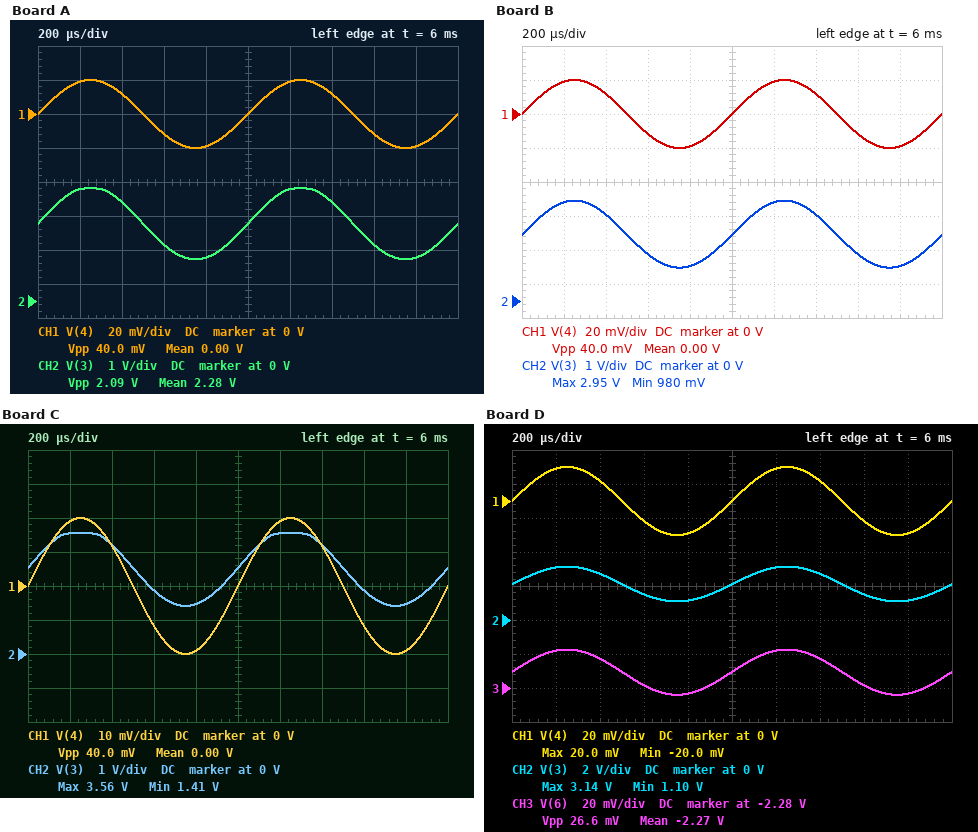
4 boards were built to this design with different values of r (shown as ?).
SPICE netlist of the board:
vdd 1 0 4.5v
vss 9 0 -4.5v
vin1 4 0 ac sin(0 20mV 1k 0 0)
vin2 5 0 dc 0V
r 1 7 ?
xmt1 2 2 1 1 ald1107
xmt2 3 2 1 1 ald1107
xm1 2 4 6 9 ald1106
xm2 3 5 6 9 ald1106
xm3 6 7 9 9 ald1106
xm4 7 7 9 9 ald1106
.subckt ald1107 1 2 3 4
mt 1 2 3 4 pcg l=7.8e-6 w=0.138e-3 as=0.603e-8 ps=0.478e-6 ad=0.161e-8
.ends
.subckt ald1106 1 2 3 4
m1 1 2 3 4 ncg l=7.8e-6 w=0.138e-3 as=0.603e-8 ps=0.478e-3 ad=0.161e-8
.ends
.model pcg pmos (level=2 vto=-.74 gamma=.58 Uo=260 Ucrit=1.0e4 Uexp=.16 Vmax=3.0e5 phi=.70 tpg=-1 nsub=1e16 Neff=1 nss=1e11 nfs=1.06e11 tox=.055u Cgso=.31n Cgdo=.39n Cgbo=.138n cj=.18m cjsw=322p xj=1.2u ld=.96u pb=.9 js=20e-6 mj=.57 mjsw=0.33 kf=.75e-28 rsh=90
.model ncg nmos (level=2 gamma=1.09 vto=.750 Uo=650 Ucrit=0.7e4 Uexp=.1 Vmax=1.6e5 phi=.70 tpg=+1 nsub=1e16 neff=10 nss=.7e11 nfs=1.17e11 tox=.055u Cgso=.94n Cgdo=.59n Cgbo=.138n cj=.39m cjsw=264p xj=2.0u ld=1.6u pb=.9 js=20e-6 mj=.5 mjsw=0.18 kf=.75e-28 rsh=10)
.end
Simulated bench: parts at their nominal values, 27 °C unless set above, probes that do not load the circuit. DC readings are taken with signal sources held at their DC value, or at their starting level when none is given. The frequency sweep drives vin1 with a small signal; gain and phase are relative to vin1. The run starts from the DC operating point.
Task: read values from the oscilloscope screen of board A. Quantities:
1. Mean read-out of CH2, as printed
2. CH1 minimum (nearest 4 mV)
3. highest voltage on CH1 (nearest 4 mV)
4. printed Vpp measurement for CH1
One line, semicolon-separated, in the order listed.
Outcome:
2.28 V; -20 mV; 20 mV; 40.0 mV
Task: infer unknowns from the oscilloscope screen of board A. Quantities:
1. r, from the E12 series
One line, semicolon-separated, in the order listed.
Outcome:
15 kΩ
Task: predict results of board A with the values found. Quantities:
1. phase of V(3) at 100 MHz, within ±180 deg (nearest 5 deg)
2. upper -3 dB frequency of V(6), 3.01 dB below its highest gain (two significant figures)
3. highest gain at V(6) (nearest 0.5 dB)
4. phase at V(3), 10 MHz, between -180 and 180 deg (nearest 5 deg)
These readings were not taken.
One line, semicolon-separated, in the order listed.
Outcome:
-140 deg; 5.5 MHz; -3.5 dB; -80 deg
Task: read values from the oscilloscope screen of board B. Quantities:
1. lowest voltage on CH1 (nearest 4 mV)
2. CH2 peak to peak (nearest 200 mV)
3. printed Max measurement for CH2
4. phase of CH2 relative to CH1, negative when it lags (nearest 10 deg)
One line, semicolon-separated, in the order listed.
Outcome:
-20 mV; 2.0 V; 2.95 V; 0 deg
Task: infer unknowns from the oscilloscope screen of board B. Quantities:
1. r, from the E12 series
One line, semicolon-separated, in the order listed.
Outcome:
10 kΩ
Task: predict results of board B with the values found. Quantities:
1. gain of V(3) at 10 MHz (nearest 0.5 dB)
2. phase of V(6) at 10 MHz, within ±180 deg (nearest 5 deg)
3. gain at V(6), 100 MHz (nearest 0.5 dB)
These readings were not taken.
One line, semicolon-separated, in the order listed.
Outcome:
25.5 dB; -20 deg; -12.5 dB
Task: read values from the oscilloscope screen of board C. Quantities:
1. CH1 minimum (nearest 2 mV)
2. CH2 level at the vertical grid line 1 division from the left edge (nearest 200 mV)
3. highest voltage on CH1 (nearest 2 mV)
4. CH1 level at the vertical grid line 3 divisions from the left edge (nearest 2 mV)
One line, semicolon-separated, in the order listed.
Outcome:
-20 mV; 3.6 V; 20 mV; -12 mV
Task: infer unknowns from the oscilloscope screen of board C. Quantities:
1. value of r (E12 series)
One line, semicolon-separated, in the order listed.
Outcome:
22 kΩ
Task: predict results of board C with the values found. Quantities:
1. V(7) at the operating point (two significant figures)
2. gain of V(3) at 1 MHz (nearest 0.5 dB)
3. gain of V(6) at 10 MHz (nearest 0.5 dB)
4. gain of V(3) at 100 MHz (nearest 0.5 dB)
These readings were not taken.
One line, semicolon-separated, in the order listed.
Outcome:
-2.8 V; 34.5 dB; -8.0 dB; -2.5 dB
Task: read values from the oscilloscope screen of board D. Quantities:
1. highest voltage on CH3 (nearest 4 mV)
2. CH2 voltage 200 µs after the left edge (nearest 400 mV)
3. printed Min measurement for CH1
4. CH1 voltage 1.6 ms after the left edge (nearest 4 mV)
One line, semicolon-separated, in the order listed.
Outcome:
-2.256 V; 3.2 V; -20.0 mV; -12 mV
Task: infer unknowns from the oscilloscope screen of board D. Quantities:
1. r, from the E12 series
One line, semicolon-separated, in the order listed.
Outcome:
12 kΩ
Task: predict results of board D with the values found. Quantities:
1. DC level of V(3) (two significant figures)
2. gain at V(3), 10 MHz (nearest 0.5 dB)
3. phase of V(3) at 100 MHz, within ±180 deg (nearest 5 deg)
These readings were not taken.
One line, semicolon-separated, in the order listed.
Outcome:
2.1 V; 25.0 dB; -135 deg
